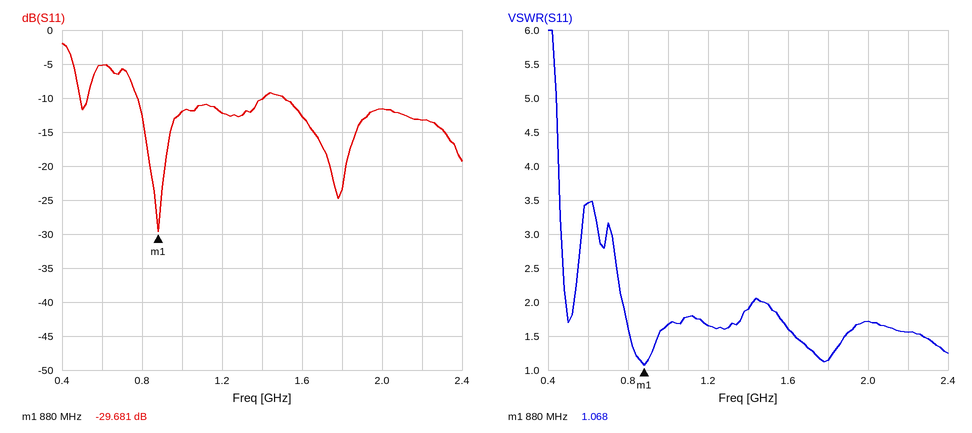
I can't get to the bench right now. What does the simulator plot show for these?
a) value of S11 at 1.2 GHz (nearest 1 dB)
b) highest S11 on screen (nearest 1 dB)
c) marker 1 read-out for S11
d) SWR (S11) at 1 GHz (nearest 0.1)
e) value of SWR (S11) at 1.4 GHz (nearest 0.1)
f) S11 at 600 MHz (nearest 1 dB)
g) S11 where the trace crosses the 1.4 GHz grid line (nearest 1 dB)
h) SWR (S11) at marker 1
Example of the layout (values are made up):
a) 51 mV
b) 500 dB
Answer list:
a) -12 dB
b) -2 dB
c) -29.681 dB
d) 1.7
e) 1.9
f) -5 dB
g) -10 dB
h) 1.068
